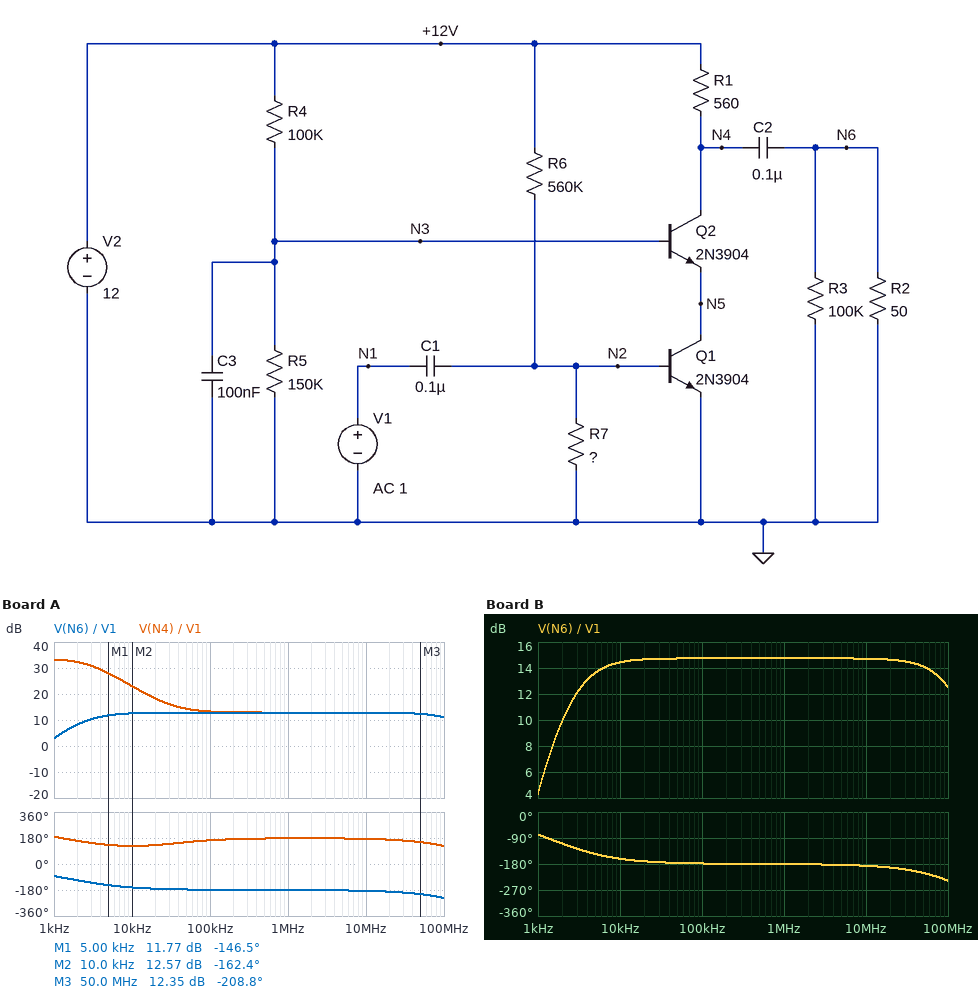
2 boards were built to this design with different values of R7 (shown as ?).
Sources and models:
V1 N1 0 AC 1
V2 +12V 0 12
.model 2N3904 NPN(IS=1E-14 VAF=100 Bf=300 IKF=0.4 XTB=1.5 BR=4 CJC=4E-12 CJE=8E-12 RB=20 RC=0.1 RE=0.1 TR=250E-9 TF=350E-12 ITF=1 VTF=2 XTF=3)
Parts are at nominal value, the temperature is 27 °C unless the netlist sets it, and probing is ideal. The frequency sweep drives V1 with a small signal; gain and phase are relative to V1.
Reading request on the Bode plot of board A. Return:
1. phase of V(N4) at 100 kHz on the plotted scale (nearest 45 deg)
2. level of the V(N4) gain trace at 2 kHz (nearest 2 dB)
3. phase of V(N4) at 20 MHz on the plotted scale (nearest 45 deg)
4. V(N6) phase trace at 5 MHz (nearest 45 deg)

180 deg
32 dB
180 deg
-180 deg
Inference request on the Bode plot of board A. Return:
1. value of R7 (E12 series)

56 kΩ
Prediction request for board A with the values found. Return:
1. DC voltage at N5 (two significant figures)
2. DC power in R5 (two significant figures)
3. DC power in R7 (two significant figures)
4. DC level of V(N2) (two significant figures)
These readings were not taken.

6.0 V
300 µW
8.2 µW
680 mV
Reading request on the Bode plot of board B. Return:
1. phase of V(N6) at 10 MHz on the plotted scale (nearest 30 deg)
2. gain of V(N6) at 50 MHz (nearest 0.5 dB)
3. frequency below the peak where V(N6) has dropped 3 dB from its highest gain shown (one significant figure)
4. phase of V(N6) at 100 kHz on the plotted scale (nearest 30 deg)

-180 deg
14.0 dB
3 kHz
-180 deg
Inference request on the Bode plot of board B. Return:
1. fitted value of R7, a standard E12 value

68 kΩ
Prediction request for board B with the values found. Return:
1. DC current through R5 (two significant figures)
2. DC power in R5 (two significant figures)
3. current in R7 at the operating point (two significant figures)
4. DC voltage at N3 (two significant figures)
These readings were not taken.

44 µA
290 µW
10 µA
6.6 V
